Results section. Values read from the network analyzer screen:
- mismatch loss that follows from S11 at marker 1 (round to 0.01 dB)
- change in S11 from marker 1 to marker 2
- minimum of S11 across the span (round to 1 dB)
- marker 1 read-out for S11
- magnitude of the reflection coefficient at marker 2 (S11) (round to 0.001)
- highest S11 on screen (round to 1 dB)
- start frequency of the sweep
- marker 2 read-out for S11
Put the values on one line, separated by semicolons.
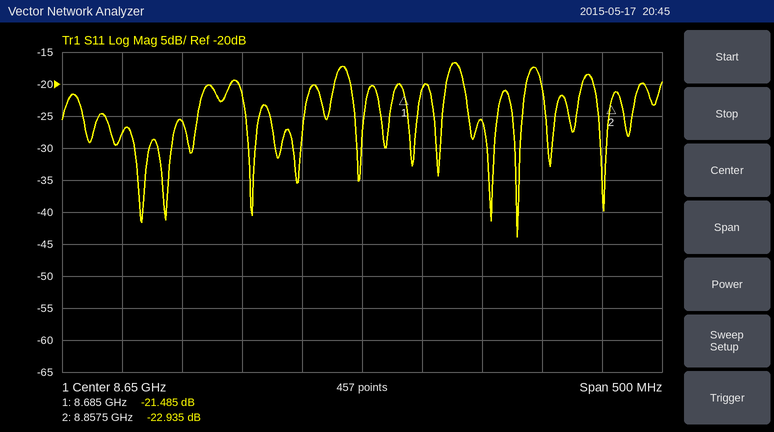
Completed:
0.03 dB; -1.450 dB; -44 dB; -21.485 dB; 0.071; -17 dB; 8.4 GHz; -22.935 dB
